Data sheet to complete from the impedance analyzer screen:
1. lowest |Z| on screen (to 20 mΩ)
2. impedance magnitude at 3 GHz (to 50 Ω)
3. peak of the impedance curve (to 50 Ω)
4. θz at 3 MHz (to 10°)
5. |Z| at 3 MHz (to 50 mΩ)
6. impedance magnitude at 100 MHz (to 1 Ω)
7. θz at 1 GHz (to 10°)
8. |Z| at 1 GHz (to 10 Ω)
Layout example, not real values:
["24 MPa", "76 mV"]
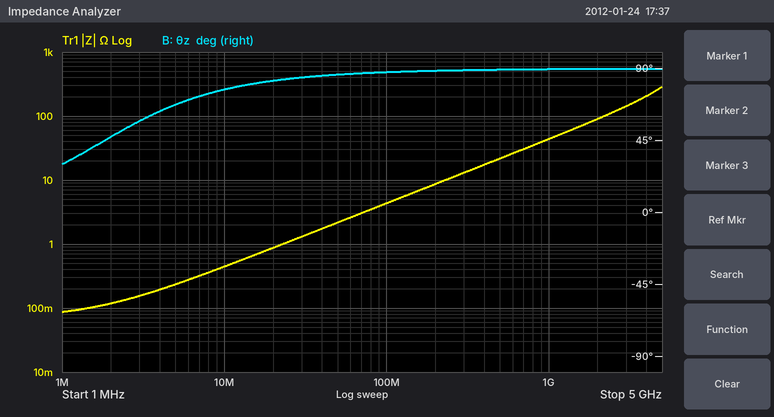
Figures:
["80 mΩ", "150 Ω", "300 Ω", "60°", "150 mΩ", "4 Ω", "90°", "40 Ω"]
